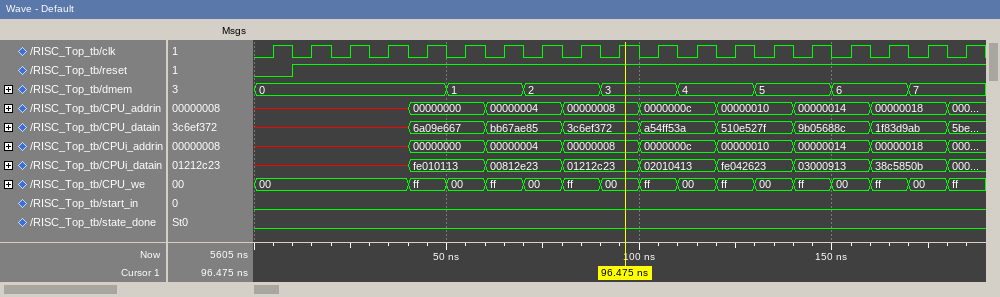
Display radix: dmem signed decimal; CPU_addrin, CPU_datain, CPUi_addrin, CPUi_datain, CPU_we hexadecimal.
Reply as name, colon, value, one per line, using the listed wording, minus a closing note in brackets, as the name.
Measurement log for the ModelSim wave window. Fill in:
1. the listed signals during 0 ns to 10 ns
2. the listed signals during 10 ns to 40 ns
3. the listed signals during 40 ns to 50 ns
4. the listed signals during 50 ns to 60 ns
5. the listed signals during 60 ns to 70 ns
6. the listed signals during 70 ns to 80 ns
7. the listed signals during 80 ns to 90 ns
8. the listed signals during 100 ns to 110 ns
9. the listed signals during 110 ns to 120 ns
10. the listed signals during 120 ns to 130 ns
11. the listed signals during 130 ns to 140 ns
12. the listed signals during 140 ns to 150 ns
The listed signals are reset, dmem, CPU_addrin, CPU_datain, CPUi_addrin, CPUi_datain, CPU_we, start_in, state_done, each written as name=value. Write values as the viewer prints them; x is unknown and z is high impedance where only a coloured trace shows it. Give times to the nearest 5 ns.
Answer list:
the listed signals during 0 ns to 10 ns: reset=0, dmem=0, CPU_addrin=x, CPU_datain=x, CPUi_addrin=x, CPUi_datain=x, CPU_we=00, start_in=0, state_done=0
the listed signals during 10 ns to 40 ns: reset=1, dmem=0, CPU_addrin=x, CPU_datain=x, CPUi_addrin=x, CPUi_datain=x, CPU_we=00, start_in=0, state_done=0
the listed signals during 40 ns to 50 ns: reset=1, dmem=0, CPU_addrin=00000000, CPU_datain=6a09e667, CPUi_addrin=00000000, CPUi_datain=fe010113, CPU_we=ff, start_in=0, state_done=0
the listed signals during 50 ns to 60 ns: reset=1, dmem=1, CPU_addrin=00000000, CPU_datain=6a09e667, CPUi_addrin=00000000, CPUi_datain=fe010113, CPU_we=00, start_in=0, state_done=0
the listed signals during 60 ns to 70 ns: reset=1, dmem=1, CPU_addrin=00000004, CPU_datain=bb67ae85, CPUi_addrin=00000004, CPUi_datain=00812e23, CPU_we=ff, start_in=0, state_done=0
the listed signals during 70 ns to 80 ns: reset=1, dmem=2, CPU_addrin=00000004, CPU_datain=bb67ae85, CPUi_addrin=00000004, CPUi_datain=00812e23, CPU_we=00, start_in=0, state_done=0
the listed signals during 80 ns to 90 ns: reset=1, dmem=2, CPU_addrin=00000008, CPU_datain=3c6ef372, CPUi_addrin=00000008, CPUi_datain=01212c23, CPU_we=ff, start_in=0, state_done=0
the listed signals during 100 ns to 110 ns: reset=1, dmem=3, CPU_addrin=0000000c, CPU_datain=a54ff53a, CPUi_addrin=0000000c, CPUi_datain=02010413, CPU_we=ff, start_in=0, state_done=0
the listed signals during 110 ns to 120 ns: reset=1, dmem=4, CPU_addrin=0000000c, CPU_datain=a54ff53a, CPUi_addrin=0000000c, CPUi_datain=02010413, CPU_we=00, start_in=0, state_done=0
the listed signals during 120 ns to 130 ns: reset=1, dmem=4, CPU_addrin=00000010, CPU_datain=510e527f, CPUi_addrin=00000010, CPUi_datain=fe042623, CPU_we=ff, start_in=0, state_done=0
the listed signals during 130 ns to 140 ns: reset=1, dmem=5, CPU_addrin=00000010, CPU_datain=510e527f, CPUi_addrin=00000010, CPUi_datain=fe042623, CPU_we=00, start_in=0, state_done=0
the listed signals during 140 ns to 150 ns: reset=1, dmem=5, CPU_addrin=00000014, CPU_datain=9b05688c, CPUi_addrin=00000014, CPUi_datain=03000913, CPU_we=ff, start_in=0, state_done=0
